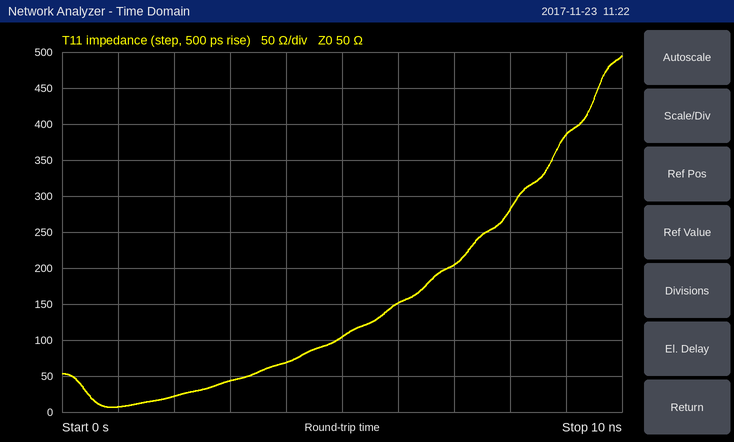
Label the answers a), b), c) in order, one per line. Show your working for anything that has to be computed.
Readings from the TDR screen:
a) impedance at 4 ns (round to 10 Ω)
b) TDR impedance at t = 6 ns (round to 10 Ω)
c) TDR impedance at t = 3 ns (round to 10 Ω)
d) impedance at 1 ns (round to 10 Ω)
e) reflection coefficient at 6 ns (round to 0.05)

a) 70 Ω
b) 150 Ω
c) 40 Ω
d) 10 Ω
e) (150 − 50)/(150 + 50) ≈ +0.50
